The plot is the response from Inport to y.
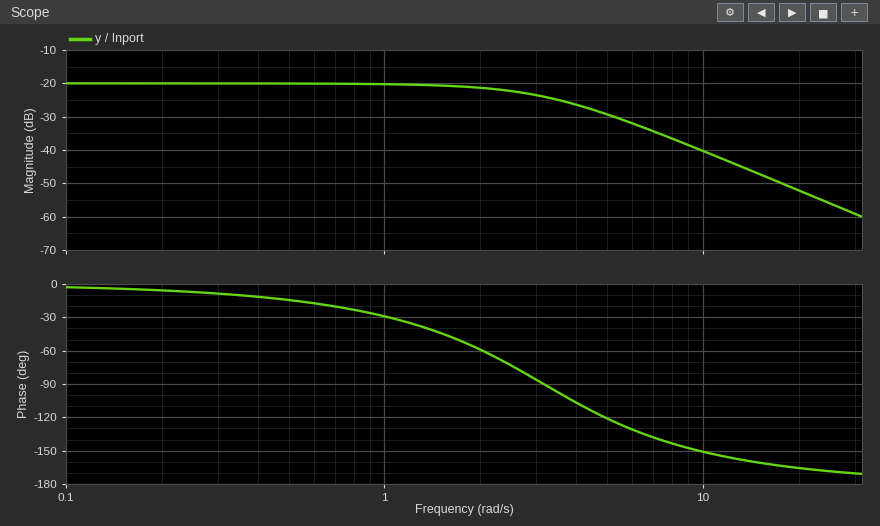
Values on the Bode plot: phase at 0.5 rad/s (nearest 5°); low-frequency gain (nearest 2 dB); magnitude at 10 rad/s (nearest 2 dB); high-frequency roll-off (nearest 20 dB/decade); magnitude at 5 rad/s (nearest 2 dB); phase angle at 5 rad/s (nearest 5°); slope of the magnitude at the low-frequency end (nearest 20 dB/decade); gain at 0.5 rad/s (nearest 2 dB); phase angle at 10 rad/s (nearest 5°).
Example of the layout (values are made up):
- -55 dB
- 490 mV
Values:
- -15°
- -20 dB
- -40 dB
- -40 dB/decade
- -30 dB
- -120°
- 0 dB/decade
- -20 dB
- -150°
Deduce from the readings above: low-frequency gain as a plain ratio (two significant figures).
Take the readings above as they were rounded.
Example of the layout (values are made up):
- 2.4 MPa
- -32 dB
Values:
- 0.10
